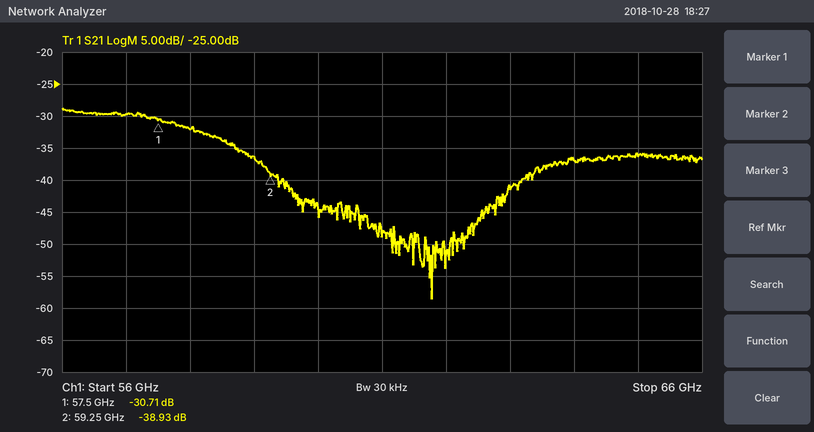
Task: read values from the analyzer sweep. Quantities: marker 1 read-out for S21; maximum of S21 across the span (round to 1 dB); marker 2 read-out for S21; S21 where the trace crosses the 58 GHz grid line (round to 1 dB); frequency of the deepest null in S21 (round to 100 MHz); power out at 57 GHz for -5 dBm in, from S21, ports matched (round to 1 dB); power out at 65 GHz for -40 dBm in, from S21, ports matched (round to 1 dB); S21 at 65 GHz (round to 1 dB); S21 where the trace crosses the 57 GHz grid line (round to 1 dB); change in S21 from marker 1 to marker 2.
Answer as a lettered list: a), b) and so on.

a) -30.71 dB
b) -29 dB
c) -38.93 dB
d) -32 dB
e) 61.8 GHz
f) -35 dBm
g) -76 dBm
h) -36 dB
i) -30 dB
j) -8.22 dB
